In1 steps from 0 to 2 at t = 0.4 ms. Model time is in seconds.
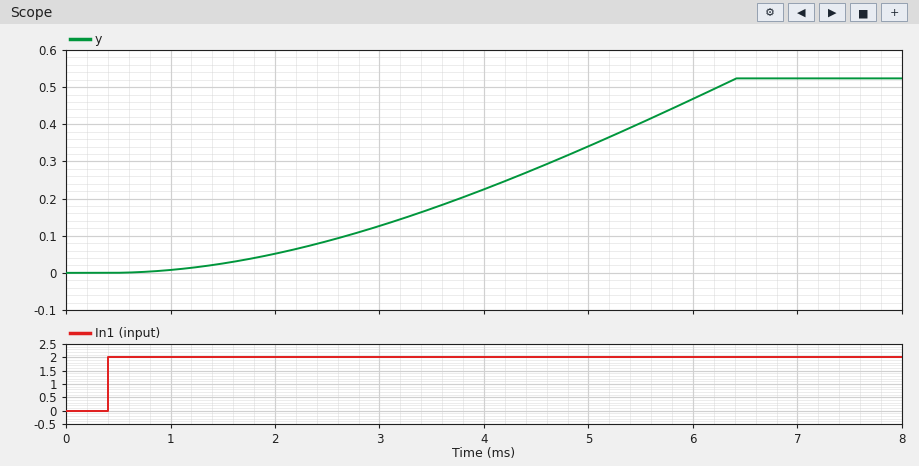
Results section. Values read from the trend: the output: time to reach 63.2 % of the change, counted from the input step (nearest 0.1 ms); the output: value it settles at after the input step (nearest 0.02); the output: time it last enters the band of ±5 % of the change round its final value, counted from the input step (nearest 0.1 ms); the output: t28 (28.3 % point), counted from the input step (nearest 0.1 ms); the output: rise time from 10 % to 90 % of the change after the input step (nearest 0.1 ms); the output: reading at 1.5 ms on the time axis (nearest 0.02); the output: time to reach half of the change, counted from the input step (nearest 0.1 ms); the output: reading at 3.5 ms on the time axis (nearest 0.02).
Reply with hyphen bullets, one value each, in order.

- 4.5 ms
- 0.52
- 5.8 ms
- 2.8 ms
- 4.0 ms
- 0.02
- 3.9 ms
- 0.18
